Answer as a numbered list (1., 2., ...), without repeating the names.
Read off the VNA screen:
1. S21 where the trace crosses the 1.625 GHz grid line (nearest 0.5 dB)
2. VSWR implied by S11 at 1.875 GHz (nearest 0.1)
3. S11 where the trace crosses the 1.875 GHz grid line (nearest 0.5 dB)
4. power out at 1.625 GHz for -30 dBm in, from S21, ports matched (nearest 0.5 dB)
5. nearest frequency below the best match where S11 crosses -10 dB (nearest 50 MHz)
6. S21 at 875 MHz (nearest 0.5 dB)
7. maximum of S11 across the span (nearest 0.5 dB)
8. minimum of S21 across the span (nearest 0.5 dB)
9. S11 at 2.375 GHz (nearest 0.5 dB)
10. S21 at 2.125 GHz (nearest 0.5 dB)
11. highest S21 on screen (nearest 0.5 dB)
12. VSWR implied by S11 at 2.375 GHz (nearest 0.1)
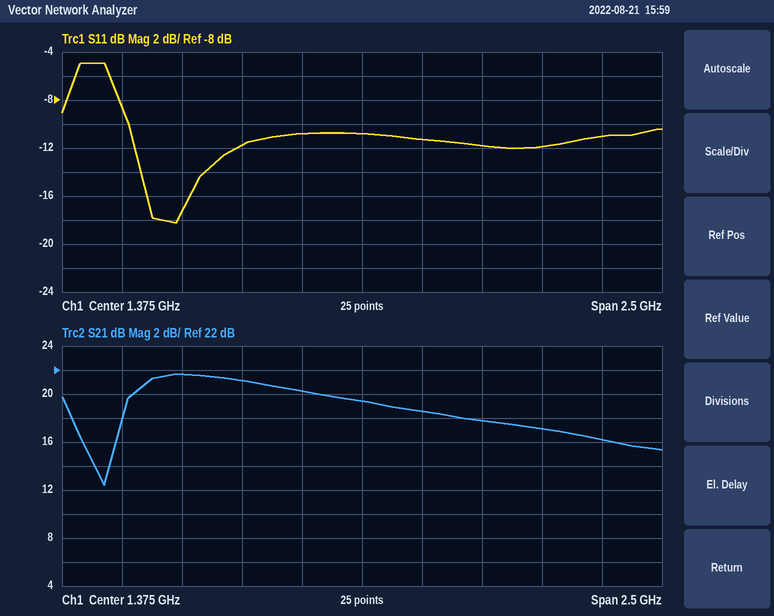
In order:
1. 18.5 dB
2. 1.7
3. -12.0 dB
4. -11.5 dBm
5. 400 MHz
6. 21.0 dB
7. -5.0 dB
8. 12.5 dB
9. -11.0 dB
10. 17.0 dB
11. 21.5 dB
12. 1.8
